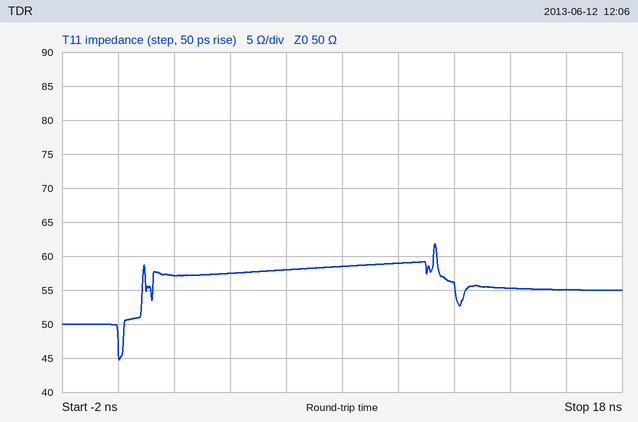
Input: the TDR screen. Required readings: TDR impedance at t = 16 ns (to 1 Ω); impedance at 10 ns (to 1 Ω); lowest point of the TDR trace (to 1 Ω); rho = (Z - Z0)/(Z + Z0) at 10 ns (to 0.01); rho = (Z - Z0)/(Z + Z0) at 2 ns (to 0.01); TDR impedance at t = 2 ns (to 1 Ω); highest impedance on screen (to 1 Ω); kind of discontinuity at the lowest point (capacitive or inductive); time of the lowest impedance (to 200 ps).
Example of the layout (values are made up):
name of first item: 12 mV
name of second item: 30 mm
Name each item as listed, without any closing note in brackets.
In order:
TDR impedance at t = 16 ns: 55 Ω
impedance at 10 ns: 59 Ω
lowest point of the TDR trace: 45 Ω
rho = (Z - Z0)/(Z + Z0) at 10 ns: +0.08
rho = (Z - Z0)/(Z + Z0) at 2 ns: +0.07
TDR impedance at t = 2 ns: 57 Ω
highest impedance on screen: 62 Ω
kind of discontinuity at the lowest point: capacitive
time of the lowest impedance: 0.0 ns
